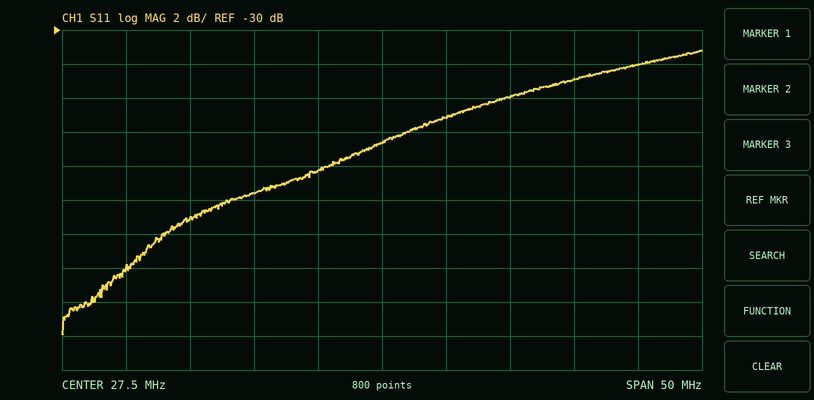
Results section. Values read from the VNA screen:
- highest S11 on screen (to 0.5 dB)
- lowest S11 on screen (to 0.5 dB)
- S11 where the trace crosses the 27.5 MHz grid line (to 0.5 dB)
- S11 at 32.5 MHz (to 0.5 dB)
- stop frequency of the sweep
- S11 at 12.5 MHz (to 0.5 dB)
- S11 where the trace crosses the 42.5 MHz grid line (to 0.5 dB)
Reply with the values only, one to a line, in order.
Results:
-31.0 dB
-48.0 dB
-36.5 dB
-35.0 dB
52.5 MHz
-41.0 dB
-33.0 dB
